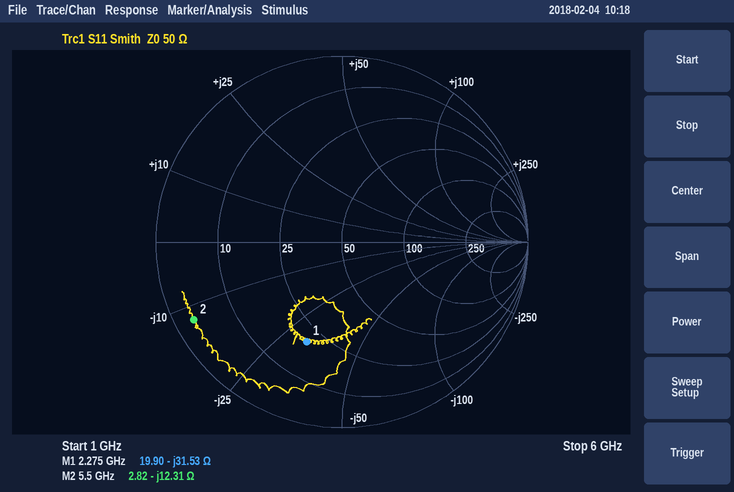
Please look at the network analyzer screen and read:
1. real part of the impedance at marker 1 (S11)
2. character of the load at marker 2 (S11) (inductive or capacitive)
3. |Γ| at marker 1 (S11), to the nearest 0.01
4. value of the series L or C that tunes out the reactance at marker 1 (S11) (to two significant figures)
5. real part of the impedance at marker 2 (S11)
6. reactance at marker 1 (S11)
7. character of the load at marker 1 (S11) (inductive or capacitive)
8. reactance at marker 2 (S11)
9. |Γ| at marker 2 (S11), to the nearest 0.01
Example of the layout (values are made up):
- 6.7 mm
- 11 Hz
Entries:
- 19.90 Ω
- capacitive
- 0.57
- 2.2 nH
- 2.82 Ω
- -31.53 Ω
- capacitive
- -12.31 Ω
- 0.90
